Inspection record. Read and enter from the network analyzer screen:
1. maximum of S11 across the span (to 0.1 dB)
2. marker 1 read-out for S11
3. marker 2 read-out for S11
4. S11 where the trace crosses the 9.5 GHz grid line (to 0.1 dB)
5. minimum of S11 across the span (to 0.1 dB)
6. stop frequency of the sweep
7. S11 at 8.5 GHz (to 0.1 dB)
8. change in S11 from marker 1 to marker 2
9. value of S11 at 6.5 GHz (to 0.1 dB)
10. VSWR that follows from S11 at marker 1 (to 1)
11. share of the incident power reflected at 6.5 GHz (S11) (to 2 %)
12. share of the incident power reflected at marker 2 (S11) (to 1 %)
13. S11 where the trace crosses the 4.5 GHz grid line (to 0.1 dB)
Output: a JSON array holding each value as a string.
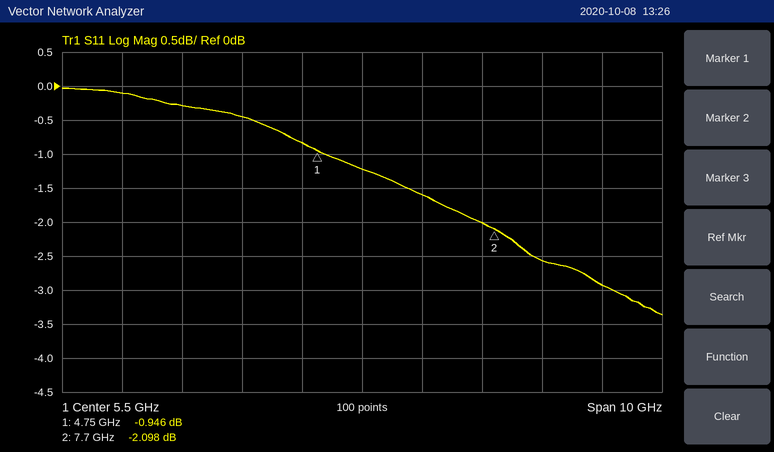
["0.0 dB", "-0.946 dB", "-2.098 dB", "-2.9 dB", "-3.4 dB", "10.5 GHz", "-2.6 dB", "-1.152 dB", "-1.6 dB", "18", "70 %", "62 %", "-0.8 dB"]
